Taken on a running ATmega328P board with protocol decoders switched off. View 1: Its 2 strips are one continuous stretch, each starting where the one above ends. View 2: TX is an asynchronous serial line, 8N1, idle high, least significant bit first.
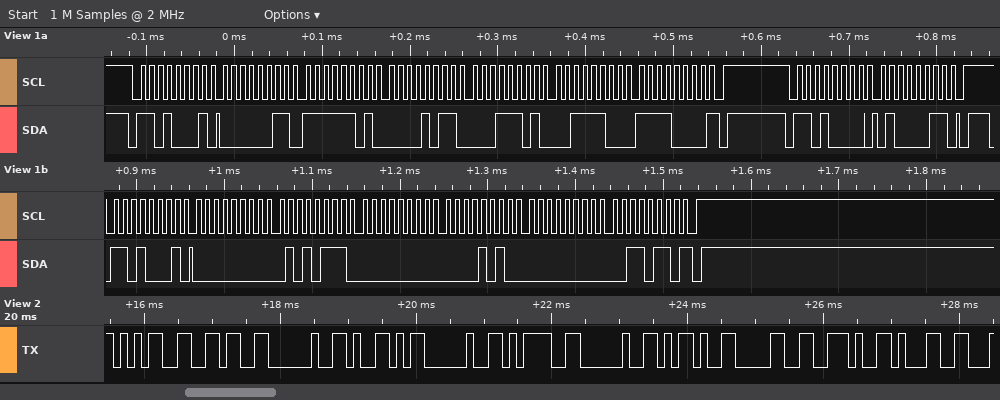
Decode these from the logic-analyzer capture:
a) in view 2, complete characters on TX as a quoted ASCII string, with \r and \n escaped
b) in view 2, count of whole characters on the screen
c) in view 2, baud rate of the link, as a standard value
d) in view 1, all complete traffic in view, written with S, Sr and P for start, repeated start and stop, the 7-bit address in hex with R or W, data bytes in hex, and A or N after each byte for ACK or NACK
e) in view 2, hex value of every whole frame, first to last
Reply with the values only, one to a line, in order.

"56 Y = -0.1"
11
9600 baud
S 68R A 03 A FD A 0B A 1D A 3C A F0 N P S 68W A 43 A P S 68R A 00 A 57 A 00 A 0A A 00 A 36 N P
0x35 0x36 0x20 0x59 0x20 0x3D 0x20 0x2D 0x30 0x2E 0x31
